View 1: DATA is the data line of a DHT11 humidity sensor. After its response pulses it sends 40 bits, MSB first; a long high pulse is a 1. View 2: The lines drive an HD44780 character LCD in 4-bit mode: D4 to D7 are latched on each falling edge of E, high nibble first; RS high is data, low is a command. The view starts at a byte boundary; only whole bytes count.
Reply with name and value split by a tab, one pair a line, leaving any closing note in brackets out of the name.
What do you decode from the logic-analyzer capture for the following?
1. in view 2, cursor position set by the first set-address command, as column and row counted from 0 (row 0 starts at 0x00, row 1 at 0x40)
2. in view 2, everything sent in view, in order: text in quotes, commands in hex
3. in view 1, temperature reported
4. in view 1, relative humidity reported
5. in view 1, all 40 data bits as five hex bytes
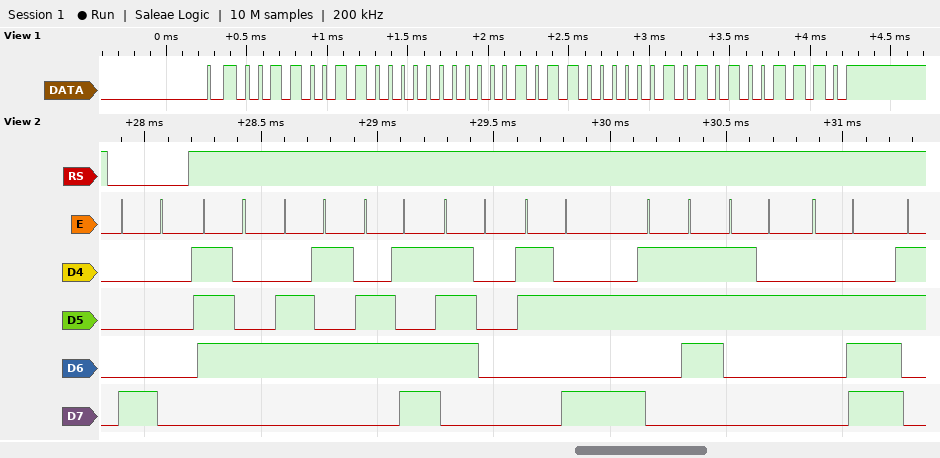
in view 2, cursor position set by the first set-address command, as column and row counted from 0	column 0, row 0
in view 2, everything sent in view, in order: text in quotes, commands in hex	0x80 "temp:72."
in view 1, temperature reported	22.5 °C
in view 1, relative humidity reported	51 %
in view 1, all 40 data bits as five hex bytes	33 00 16 05 4E
